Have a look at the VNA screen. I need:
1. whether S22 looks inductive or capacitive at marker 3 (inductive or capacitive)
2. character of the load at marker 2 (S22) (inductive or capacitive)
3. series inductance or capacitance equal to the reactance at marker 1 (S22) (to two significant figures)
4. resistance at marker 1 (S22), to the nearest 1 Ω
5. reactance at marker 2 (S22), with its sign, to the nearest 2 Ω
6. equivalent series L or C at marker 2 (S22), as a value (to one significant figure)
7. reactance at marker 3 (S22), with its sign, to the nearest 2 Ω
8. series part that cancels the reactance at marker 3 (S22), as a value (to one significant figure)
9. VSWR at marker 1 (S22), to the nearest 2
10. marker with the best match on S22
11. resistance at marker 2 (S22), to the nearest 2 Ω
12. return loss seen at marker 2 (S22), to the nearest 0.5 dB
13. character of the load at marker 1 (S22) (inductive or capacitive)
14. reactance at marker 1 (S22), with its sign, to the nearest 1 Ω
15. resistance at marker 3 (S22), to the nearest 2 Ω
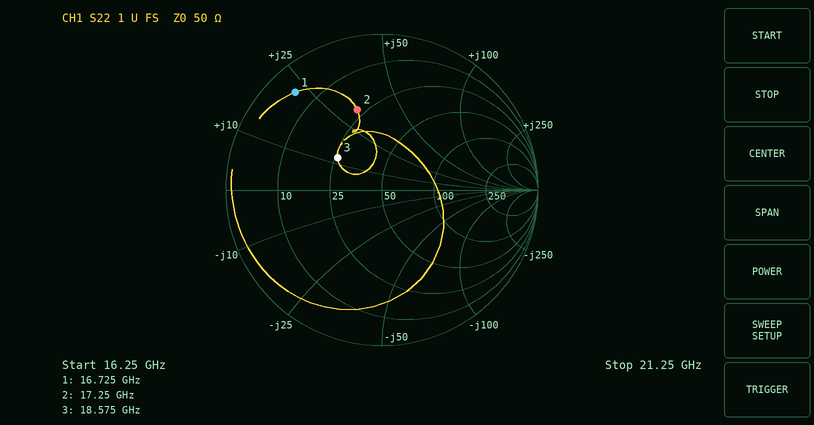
inductive
inductive
210 pH
5 Ω
+32 Ω
300 pH
+12 Ω
700 fF
12
marker 3
22 Ω
5.5 dB
inductive
+22 Ω
26 Ω
